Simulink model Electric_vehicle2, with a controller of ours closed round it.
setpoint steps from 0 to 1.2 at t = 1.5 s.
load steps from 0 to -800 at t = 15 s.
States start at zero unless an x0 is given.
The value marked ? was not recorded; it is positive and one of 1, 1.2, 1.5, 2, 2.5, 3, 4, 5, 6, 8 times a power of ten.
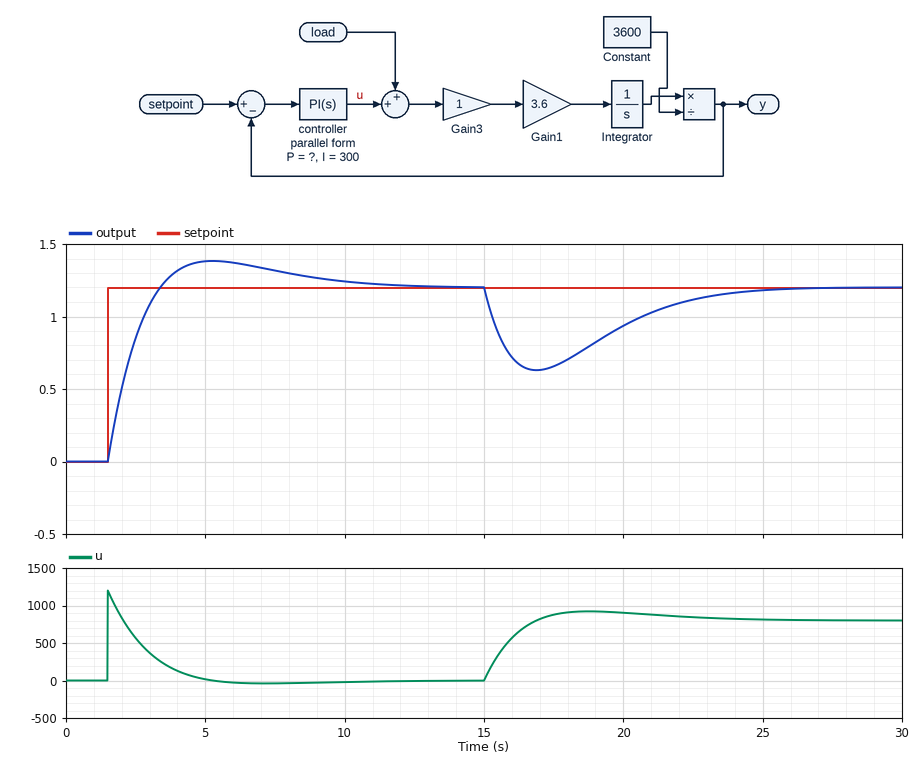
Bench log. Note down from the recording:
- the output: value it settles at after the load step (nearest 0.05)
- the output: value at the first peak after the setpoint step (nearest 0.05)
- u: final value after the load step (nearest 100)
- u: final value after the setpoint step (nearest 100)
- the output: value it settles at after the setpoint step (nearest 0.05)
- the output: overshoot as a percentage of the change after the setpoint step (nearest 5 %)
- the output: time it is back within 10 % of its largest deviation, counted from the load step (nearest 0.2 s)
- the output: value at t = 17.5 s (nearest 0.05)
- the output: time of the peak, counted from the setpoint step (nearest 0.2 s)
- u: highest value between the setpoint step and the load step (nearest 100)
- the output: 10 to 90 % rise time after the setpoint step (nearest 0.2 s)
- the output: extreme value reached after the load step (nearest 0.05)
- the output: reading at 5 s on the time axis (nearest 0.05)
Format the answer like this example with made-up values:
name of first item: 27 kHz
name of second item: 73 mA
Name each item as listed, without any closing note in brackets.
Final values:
the output: value it settles at after the load step: 1.20
the output: value at the first peak after the setpoint step: 1.40
u: final value after the load step: 800
u: final value after the setpoint step: 0
the output: value it settles at after the setpoint step: 1.20
the output: overshoot as a percentage of the change after the setpoint step: 15 %
the output: time it is back within 10 % of its largest deviation, counted from the load step: 8.2 s
the output: value at t = 17.5 s: 0.65
the output: time of the peak, counted from the setpoint step: 3.8 s
u: highest value between the setpoint step and the load step: 1200
the output: 10 to 90 % rise time after the setpoint step: 1.4 s
the output: extreme value reached after the load step: 0.65
the output: reading at 5 s on the time axis: 1.40
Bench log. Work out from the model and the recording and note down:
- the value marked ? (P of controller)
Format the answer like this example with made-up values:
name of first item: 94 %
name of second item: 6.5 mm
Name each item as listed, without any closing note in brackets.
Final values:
the value marked ?: 1000
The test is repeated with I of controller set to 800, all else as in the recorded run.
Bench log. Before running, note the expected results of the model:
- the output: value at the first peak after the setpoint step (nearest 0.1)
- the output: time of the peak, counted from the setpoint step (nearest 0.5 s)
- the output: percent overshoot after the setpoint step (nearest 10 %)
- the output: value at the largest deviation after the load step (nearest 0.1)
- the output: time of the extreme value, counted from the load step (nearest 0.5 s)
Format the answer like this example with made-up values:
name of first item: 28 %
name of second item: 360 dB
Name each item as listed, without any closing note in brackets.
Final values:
the output: value at the first peak after the setpoint step: 1.5
the output: time of the peak, counted from the setpoint step: 2.5 s
the output: percent overshoot after the setpoint step: 30 %
the output: value at the largest deviation after the load step: 0.7
the output: time of the extreme value, counted from the load step: 1.5 s
